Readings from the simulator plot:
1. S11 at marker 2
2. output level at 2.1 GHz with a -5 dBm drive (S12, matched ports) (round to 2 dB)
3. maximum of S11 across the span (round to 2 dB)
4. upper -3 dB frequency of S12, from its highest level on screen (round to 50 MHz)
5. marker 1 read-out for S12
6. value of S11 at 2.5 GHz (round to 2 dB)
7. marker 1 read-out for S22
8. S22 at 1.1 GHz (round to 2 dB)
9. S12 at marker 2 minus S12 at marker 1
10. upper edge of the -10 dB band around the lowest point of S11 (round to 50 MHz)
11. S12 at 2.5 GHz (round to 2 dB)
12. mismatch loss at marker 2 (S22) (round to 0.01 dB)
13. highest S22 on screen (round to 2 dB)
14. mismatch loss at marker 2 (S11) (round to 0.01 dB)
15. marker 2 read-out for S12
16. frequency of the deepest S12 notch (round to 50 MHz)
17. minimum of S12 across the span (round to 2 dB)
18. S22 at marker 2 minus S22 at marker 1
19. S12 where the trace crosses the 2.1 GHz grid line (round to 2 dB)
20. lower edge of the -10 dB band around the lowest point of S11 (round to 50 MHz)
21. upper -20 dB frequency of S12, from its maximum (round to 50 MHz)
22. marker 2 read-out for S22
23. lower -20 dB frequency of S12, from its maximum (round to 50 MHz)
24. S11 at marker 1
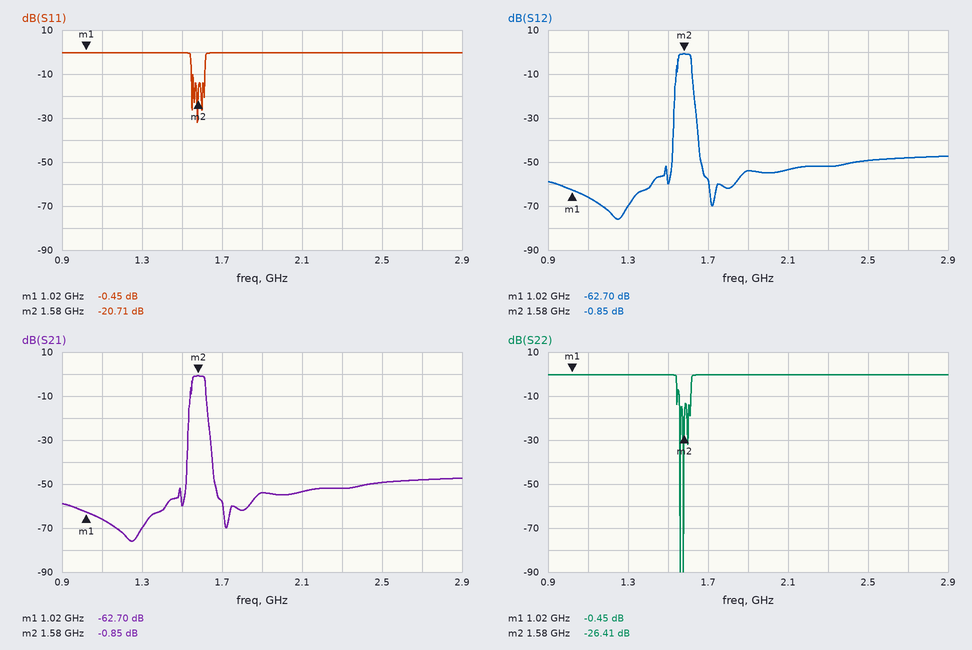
-20.71 dB
-58 dBm
0 dB
1.60 GHz
-62.70 dB
0 dB
-0.45 dB
0 dB
61.85 dB
1.60 GHz
-50 dB
0.01 dB
0 dB
0.04 dB
-0.85 dB
1.25 GHz
-76 dB
-25.96 dB
-54 dB
1.55 GHz
1.65 GHz
-26.41 dB
1.55 GHz
-0.45 dB
